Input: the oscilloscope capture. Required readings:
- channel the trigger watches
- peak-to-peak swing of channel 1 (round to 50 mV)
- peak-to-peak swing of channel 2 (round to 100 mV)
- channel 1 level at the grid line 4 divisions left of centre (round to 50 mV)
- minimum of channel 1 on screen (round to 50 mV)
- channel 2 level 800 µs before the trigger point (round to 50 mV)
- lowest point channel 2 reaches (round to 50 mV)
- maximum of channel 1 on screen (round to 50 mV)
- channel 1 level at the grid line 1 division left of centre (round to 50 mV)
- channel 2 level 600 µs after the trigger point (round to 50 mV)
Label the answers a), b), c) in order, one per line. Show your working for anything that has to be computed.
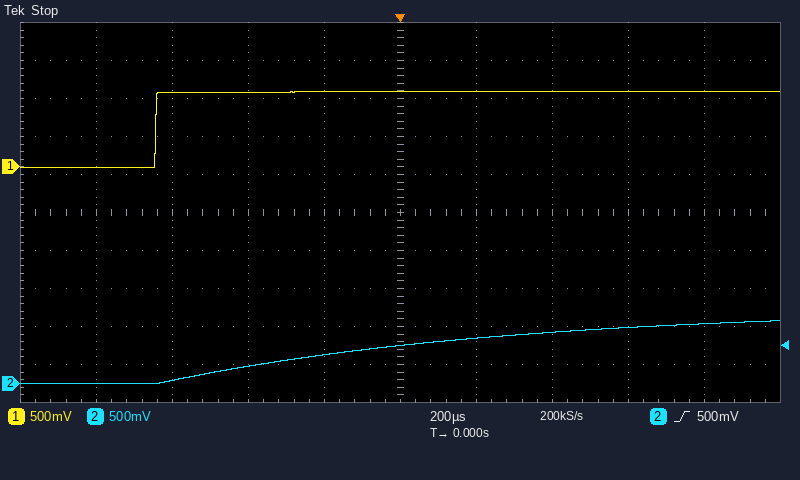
a) channel 2
b) 1.00 V − (0 mV) = 1.00 V
c) 800 mV
d) 0 mV
e) 0 mV
f) 0 mV
g) 0 mV
h) 1.00 V
i) 1.00 V
j) 750 mV
